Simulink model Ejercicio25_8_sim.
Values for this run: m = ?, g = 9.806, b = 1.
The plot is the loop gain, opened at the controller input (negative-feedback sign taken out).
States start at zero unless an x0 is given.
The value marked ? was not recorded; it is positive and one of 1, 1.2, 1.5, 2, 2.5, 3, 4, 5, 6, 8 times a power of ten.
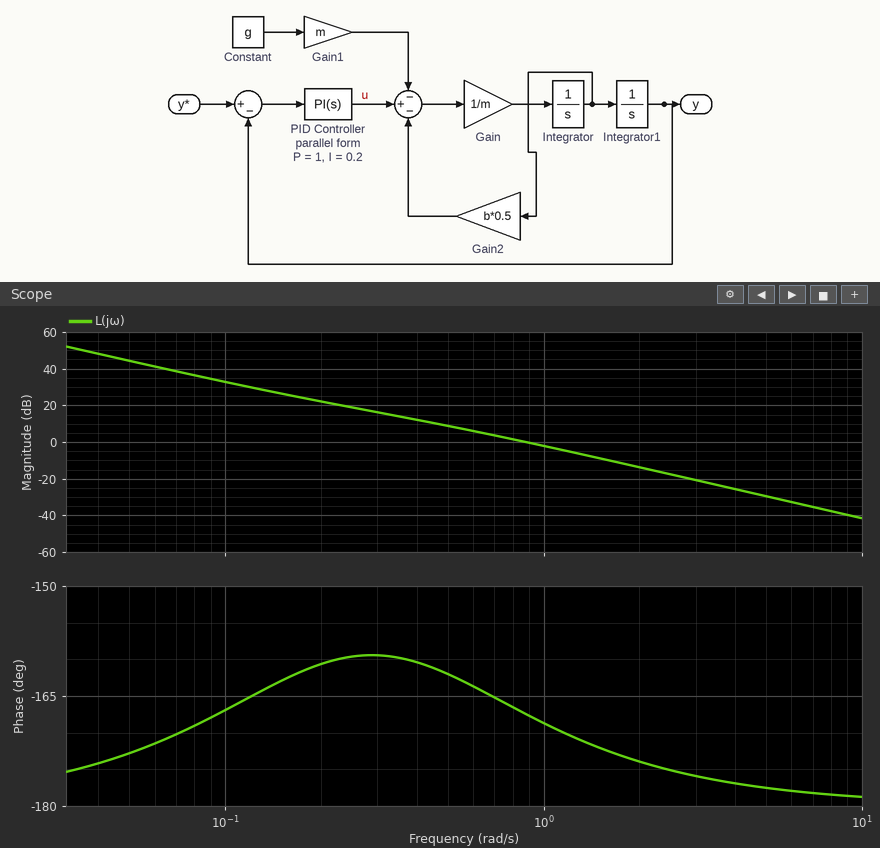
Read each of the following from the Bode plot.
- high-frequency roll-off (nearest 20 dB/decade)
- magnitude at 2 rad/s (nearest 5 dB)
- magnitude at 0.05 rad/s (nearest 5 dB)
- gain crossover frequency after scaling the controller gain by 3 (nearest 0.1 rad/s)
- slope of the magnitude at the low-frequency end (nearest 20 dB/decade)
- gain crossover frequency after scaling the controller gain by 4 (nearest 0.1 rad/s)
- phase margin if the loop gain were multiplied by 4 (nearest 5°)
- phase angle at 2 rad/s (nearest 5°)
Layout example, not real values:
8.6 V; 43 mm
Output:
-40 dB/decade; -15 dB; 45 dB; 1.6 rad/s; -40 dB/decade; 1.8 rad/s; 5°; -175°
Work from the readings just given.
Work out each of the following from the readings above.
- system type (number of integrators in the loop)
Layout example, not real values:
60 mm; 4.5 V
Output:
2
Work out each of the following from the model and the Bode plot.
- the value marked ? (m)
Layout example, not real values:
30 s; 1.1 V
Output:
1.2
